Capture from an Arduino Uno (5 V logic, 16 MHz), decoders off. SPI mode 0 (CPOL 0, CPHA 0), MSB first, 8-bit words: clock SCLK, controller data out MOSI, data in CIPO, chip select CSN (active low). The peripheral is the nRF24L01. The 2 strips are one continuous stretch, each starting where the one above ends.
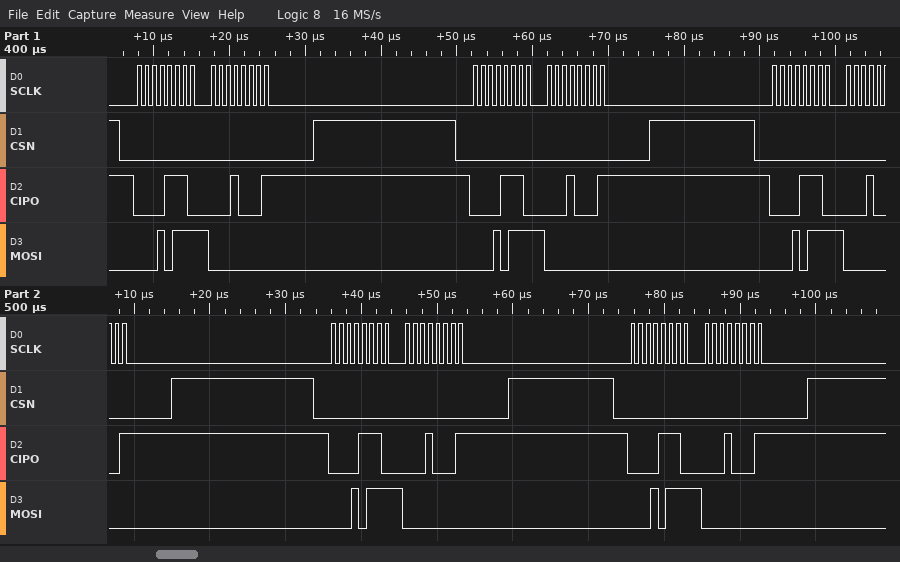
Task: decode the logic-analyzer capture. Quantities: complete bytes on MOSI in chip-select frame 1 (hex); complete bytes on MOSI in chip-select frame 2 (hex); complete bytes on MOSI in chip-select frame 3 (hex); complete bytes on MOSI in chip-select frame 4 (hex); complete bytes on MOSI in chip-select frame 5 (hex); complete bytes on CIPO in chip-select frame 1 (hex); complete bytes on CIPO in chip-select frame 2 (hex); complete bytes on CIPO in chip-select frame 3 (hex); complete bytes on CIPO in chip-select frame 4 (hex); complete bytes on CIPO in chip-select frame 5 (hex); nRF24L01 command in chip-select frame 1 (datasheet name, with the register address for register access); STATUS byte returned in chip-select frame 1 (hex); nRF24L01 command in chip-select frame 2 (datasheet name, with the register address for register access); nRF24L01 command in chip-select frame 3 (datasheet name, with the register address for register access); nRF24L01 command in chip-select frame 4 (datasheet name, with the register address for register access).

0x17 0x00
0x17 0x00
0x17 0x00
0x17 0x00
0x17 0x00
0x0E 0x11
0x0E 0x11
0x0E 0x11
0x0E 0x11
0x0E 0x11
R_REGISTER 0x17
0x0E
R_REGISTER 0x17
R_REGISTER 0x17
R_REGISTER 0x17
